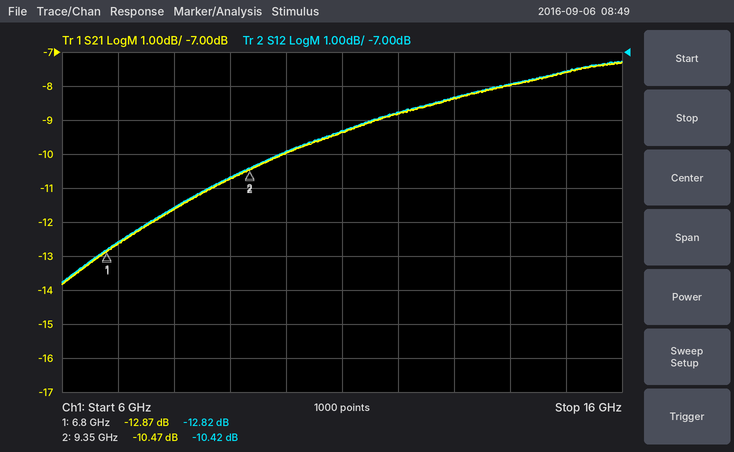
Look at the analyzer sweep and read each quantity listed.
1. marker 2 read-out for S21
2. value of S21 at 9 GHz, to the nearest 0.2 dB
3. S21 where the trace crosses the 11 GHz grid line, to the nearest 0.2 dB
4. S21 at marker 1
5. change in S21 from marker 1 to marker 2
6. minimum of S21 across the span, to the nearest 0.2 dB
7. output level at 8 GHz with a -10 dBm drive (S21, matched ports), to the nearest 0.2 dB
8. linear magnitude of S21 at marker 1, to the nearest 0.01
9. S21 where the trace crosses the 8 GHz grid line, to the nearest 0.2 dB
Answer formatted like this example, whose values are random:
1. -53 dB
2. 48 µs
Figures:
1. -10.47 dB
2. -10.8 dB
3. -9.4 dB
4. -12.87 dB
5. 2.40 dB
6. -13.8 dB
7. -21.6 dBm
8. 0.23
9. -11.6 dB
